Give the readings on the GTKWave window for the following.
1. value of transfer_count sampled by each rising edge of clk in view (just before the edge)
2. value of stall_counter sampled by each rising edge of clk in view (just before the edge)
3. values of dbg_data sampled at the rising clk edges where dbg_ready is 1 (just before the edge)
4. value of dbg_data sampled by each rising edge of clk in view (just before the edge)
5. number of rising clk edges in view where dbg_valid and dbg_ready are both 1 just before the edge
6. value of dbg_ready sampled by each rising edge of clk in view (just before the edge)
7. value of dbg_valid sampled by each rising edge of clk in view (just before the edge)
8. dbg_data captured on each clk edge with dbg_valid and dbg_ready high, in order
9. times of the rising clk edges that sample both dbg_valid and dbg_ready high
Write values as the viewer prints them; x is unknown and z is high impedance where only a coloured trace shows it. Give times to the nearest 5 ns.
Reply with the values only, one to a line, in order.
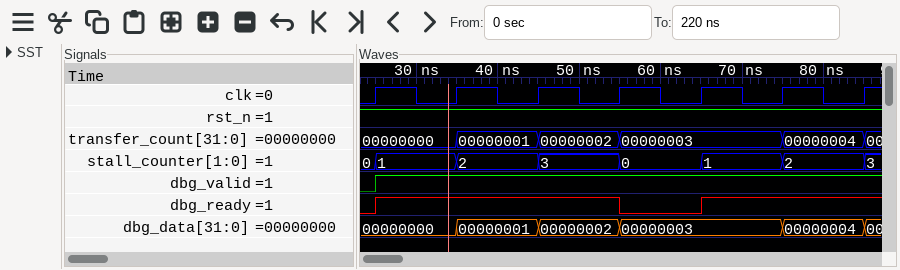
00000000, 00000000, 00000001, 00000002, 00000003, 00000003, 00000004
0, 1, 2, 3, 0, 1, 2
00000000, 00000001, 00000002, 00000003, 00000004
00000000, 00000000, 00000001, 00000002, 00000003, 00000003, 00000004
5
0 1 1 1 0 1 1
0 1 1 1 1 1 1
00000000, 00000001, 00000002, 00000003, 00000004
35 ns, 45 ns, 55 ns, 75 ns, 85 ns
